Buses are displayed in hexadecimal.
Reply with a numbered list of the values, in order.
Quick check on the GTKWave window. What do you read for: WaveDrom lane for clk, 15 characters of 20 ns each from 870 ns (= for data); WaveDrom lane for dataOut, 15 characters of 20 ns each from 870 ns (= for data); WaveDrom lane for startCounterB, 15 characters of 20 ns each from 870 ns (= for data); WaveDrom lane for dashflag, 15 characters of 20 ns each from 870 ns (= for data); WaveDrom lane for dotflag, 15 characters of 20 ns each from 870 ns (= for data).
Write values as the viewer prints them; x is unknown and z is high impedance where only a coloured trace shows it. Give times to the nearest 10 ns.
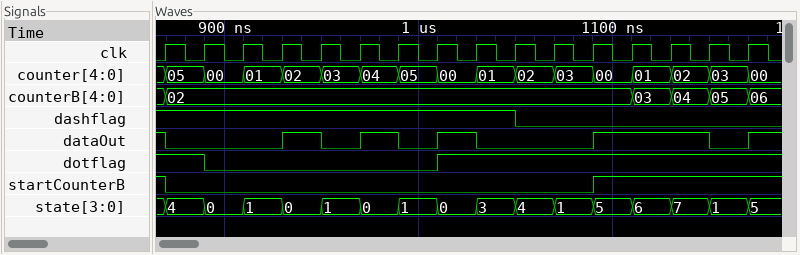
1. {name: 'clk', wave: 'p..............'}
2. {name: 'dataOut', wave: '0..101010..1..0'}
3. {name: 'startCounterB', wave: '0..........1...'}
4. {name: 'dashflag', wave: '1........0.....'}
5. {name: 'dotflag', wave: '10.....1.......'}
